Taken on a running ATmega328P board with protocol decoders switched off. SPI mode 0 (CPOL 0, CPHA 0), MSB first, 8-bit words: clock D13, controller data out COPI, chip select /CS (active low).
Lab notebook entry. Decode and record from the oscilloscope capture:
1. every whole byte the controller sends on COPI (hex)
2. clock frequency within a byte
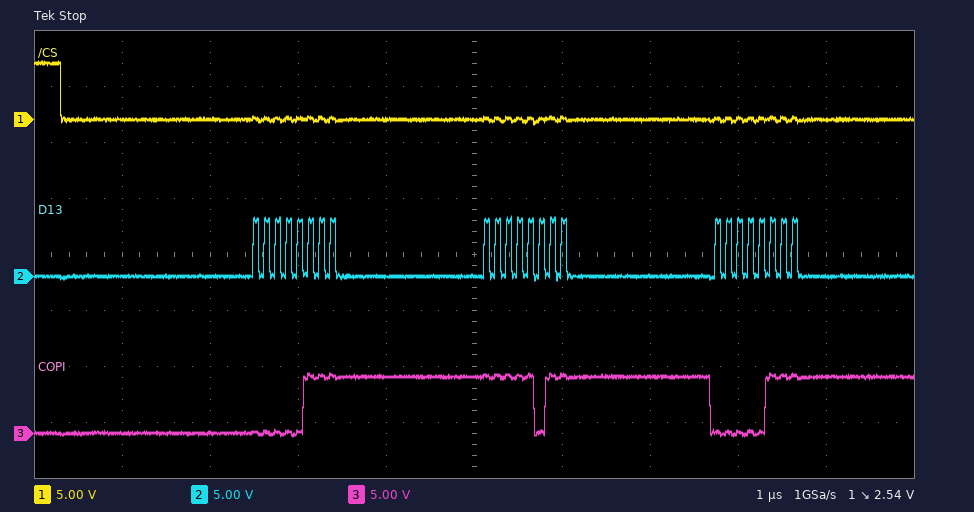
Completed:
07 FB 07
8 MHz
